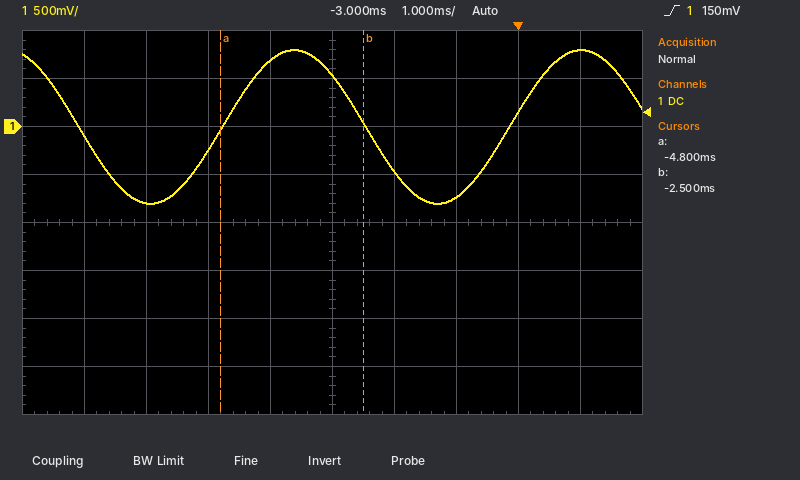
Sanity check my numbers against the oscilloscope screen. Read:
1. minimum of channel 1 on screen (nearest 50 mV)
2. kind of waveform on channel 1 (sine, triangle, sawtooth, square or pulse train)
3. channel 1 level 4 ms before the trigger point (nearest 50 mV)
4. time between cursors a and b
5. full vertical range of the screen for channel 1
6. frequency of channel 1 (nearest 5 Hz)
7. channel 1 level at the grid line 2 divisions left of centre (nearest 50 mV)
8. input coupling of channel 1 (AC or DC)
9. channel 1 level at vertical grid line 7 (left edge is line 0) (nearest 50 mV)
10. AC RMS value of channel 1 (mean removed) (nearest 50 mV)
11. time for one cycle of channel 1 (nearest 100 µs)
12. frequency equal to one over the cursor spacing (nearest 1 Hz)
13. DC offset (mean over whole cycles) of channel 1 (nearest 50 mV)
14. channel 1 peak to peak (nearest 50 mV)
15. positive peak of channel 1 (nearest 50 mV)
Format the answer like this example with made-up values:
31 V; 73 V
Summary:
-800 mV; sine; 700 mV; 2.3 ms; 4 V; 215 Hz; -250 mV; DC; -750 mV; 550 mV; 4.6 ms; 435 Hz; 0 mV; 1.60 V; 800 mV
